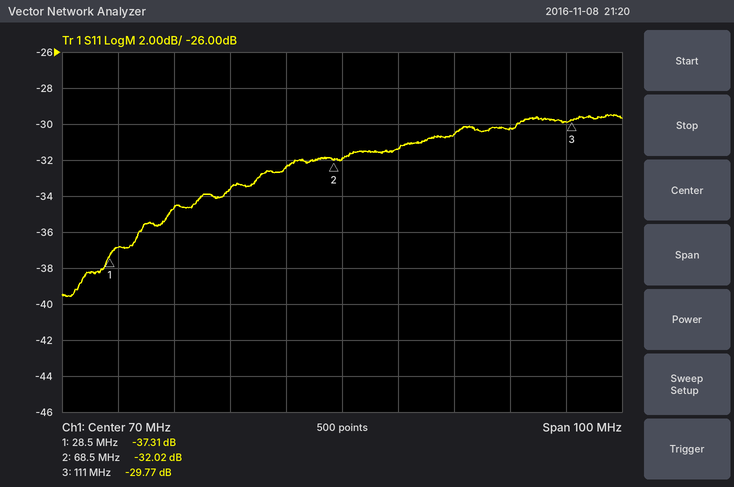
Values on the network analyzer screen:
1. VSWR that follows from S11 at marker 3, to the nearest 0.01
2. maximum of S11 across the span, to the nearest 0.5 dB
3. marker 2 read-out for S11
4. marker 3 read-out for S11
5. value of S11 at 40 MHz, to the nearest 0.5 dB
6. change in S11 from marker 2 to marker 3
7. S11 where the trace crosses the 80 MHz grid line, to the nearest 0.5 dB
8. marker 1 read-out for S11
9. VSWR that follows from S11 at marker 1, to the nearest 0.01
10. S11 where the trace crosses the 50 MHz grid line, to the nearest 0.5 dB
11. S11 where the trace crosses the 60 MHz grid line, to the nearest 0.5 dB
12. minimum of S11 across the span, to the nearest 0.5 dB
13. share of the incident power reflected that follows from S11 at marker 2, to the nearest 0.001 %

1.07
-29.5 dB
-32.02 dB
-29.77 dB
-34.5 dB
2.25 dB
-31.5 dB
-37.31 dB
1.03
-33.5 dB
-32.5 dB
-39.5 dB
0.063 %
